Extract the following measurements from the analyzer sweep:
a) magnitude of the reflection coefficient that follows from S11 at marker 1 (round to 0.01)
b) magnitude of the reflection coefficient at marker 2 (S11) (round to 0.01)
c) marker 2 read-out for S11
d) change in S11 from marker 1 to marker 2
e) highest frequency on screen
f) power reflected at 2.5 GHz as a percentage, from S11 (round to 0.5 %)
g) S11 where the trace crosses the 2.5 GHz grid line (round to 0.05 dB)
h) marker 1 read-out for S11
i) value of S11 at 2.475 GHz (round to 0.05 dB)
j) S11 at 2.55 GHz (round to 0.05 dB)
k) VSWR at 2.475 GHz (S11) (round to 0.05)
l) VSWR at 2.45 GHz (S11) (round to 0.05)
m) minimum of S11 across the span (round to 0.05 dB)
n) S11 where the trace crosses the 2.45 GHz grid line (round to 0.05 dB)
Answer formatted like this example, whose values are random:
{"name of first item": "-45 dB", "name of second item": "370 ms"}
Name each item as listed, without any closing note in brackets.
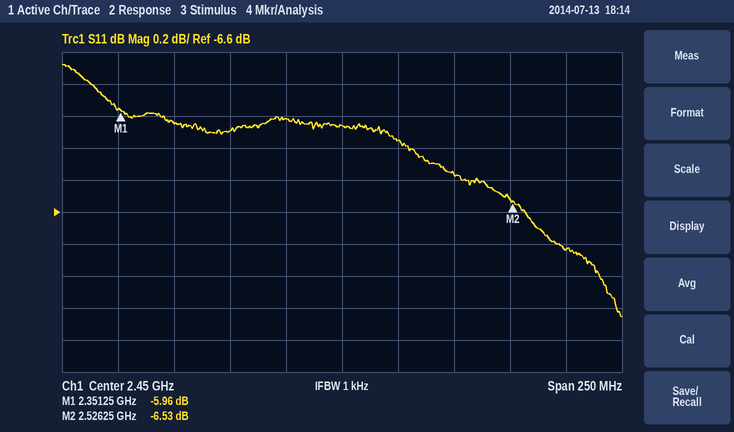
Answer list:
{"magnitude of the reflection coefficient that follows from S11 at marker 1": "0.50", "magnitude of the reflection coefficient at marker 2 (S11)": "0.47", "marker 2 read-out for S11": "-6.53 dB", "change in S11 from marker 1 to marker 2": "-0.57 dB", "highest frequency on screen": "2.575 GHz", "power reflected at 2.5 GHz as a percentage, from S11": "23.0 %", "S11 where the trace crosses the 2.5 GHz grid line": "-6.35 dB", "marker 1 read-out for S11": "-5.96 dB", "value of S11 at 2.475 GHz": "-6.15 dB", "S11 at 2.55 GHz": "-6.85 dB", "VSWR at 2.475 GHz (S11)": "2.95", "VSWR at 2.45 GHz (S11)": "3.00", "minimum of S11 across the span": "-7.25 dB", "S11 where the trace crosses the 2.45 GHz grid line": "-6.05 dB"}
